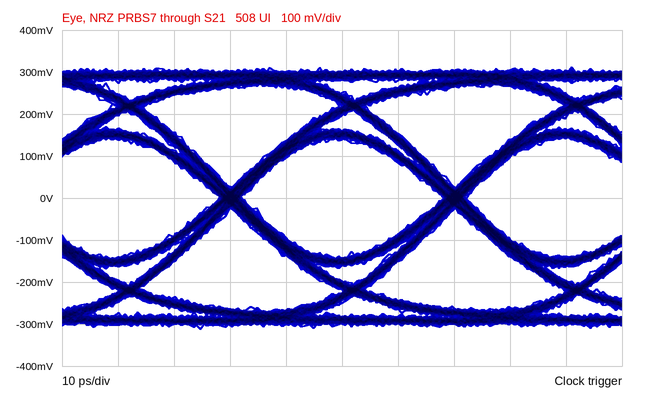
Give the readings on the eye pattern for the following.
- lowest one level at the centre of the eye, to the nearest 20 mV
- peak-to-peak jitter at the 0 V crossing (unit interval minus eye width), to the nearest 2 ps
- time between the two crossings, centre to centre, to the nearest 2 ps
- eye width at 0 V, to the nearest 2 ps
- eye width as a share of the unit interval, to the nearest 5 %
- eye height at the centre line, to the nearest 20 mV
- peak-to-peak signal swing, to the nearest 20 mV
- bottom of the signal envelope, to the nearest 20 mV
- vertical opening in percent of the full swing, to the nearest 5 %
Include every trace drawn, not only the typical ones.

140 mV
4 ps
40 ps
36 ps
90 %
280 mV
620 mV
-320 mV
45 %
